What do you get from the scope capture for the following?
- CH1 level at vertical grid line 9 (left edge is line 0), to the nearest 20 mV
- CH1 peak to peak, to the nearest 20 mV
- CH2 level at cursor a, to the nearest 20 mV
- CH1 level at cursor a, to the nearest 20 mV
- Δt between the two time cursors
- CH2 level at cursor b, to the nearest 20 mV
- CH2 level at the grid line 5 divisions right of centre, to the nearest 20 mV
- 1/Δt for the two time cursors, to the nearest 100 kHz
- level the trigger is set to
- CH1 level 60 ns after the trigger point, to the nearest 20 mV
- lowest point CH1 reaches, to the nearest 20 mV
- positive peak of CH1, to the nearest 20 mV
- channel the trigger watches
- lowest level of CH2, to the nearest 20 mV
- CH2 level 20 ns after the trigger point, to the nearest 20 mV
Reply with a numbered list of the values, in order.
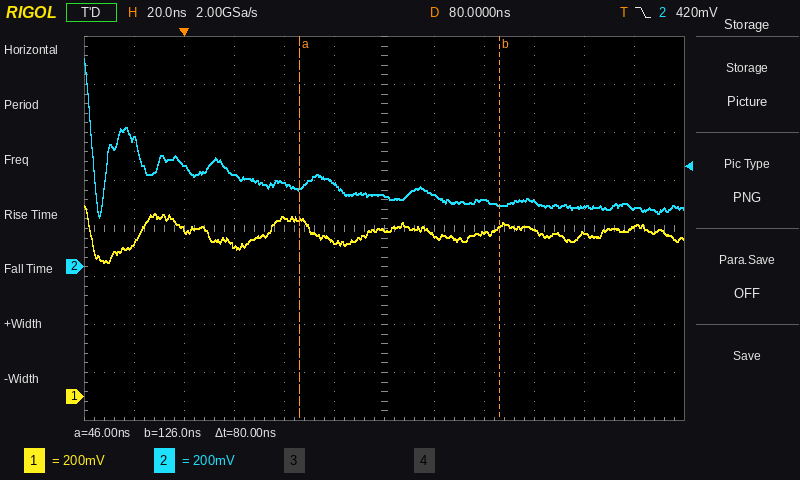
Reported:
1. 700 mV
2. 240 mV
3. 320 mV
4. 740 mV
5. 80 ns
6. 260 mV
7. 240 mV
8. 12.5 MHz
9. 420 mV
10. 640 mV
11. 560 mV
12. 800 mV
13. CH2
14. 200 mV
15. 380 mV
